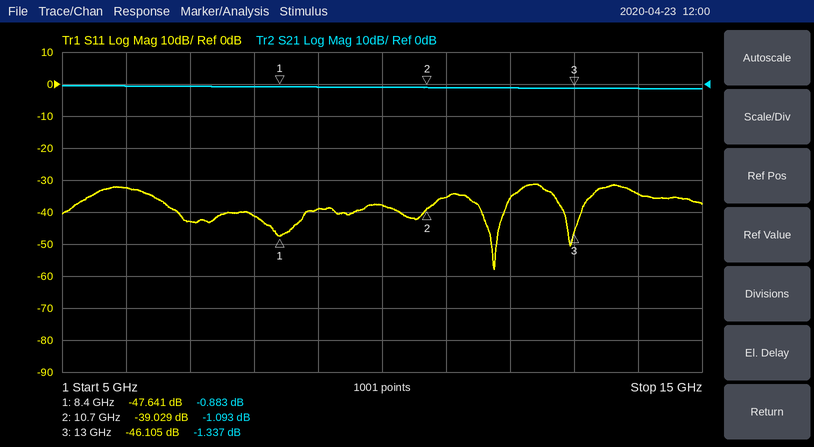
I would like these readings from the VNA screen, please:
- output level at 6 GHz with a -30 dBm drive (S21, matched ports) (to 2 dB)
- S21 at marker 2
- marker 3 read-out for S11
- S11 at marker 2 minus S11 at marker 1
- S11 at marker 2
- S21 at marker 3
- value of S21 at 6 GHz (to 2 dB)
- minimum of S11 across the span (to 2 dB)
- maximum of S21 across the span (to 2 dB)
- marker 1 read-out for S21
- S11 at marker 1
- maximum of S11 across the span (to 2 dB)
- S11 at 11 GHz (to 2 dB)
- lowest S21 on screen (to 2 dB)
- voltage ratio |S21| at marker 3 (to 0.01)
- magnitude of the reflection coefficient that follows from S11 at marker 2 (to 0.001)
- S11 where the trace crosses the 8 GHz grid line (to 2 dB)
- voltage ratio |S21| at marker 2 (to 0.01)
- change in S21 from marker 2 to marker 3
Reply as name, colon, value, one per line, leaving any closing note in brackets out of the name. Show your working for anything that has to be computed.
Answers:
output level at 6 GHz with a -30 dBm drive (S21, matched ports): -30 dBm + (0 dB) = -30 dBm
S21 at marker 2: -1.093 dB
marker 3 read-out for S11: -46.105 dB
S11 at marker 2 minus S11 at marker 1: -39.029 − (-47.641) = 8.612 dB
S11 at marker 2: -39.029 dB
S21 at marker 3: -1.337 dB
value of S21 at 6 GHz: 0 dB
minimum of S11 across the span: -58 dB
maximum of S21 across the span: 0 dB
marker 1 read-out for S21: -0.883 dB
S11 at marker 1: -47.641 dB
maximum of S11 across the span: -32 dB
S11 at 11 GHz: -36 dB
lowest S21 on screen: -2 dB
voltage ratio |S21| at marker 3: 10^(-1.337/20) ≈ 0.86
magnitude of the reflection coefficient that follows from S11 at marker 2: 10^(-39.029/20) ≈ 0.011
S11 where the trace crosses the 8 GHz grid line: -42 dB
voltage ratio |S21| at marker 2: 10^(-1.093/20) ≈ 0.88
change in S21 from marker 2 to marker 3: -1.337 − (-1.093) = -0.244 dB
